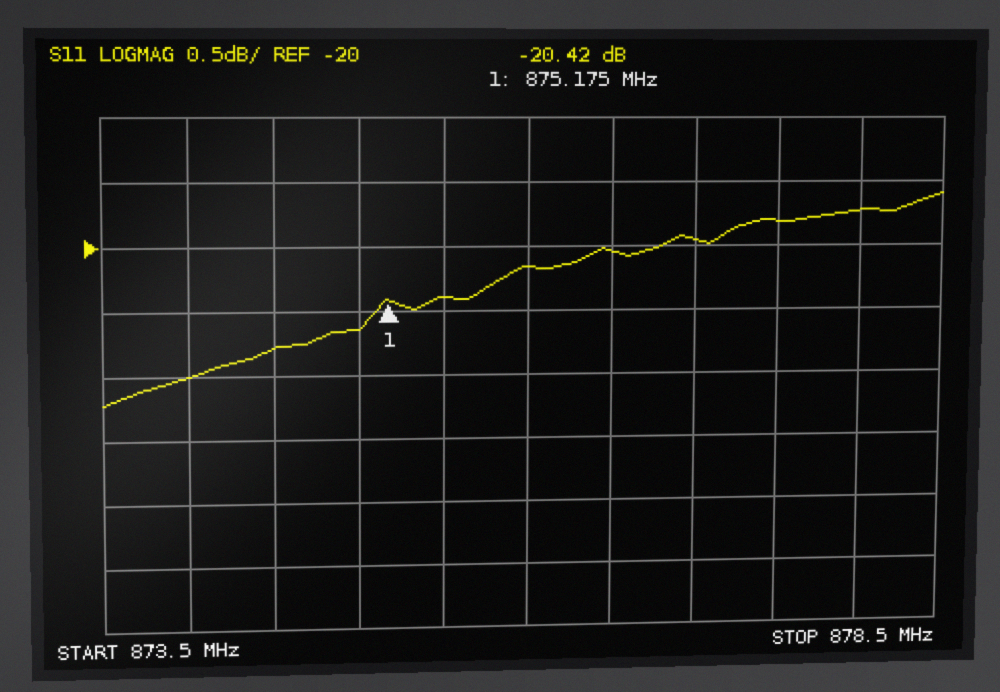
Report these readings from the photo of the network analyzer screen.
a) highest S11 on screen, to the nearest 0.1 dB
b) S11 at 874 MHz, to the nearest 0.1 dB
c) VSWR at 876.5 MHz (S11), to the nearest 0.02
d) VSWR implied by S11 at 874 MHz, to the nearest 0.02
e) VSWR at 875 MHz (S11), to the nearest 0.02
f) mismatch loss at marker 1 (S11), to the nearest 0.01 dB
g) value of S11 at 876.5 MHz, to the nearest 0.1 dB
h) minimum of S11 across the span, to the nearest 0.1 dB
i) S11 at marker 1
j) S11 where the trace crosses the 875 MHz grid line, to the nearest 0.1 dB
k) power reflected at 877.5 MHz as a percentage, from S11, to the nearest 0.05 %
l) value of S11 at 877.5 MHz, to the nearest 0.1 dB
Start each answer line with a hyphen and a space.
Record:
- -19.6 dB
- -21.0 dB
- 1.22
- 1.20
- 1.20
- 0.04 dB
- -20.0 dB
- -21.2 dB
- -20.42 dB
- -20.6 dB
- 1.05 %
- -19.8 dB
